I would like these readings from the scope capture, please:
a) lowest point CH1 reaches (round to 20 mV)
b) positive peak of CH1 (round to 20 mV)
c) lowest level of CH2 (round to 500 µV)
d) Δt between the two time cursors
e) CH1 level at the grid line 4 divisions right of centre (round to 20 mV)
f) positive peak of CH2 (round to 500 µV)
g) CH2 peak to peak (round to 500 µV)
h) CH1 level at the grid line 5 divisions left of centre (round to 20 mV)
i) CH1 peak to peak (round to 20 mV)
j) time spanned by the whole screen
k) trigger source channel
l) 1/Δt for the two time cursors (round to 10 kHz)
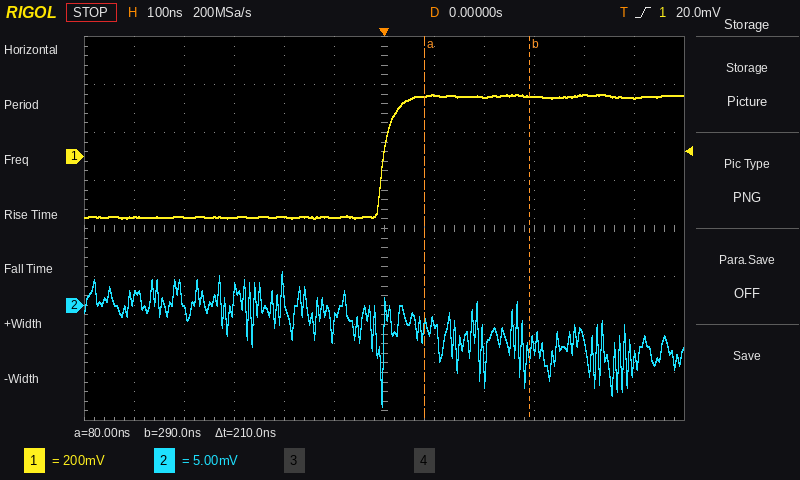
-260 mV
260 mV
-10.5 mV
210 ns
260 mV
3.5 mV
14.0 mV
-260 mV
520 mV
1.2 µs
CH1
4.76 MHz
